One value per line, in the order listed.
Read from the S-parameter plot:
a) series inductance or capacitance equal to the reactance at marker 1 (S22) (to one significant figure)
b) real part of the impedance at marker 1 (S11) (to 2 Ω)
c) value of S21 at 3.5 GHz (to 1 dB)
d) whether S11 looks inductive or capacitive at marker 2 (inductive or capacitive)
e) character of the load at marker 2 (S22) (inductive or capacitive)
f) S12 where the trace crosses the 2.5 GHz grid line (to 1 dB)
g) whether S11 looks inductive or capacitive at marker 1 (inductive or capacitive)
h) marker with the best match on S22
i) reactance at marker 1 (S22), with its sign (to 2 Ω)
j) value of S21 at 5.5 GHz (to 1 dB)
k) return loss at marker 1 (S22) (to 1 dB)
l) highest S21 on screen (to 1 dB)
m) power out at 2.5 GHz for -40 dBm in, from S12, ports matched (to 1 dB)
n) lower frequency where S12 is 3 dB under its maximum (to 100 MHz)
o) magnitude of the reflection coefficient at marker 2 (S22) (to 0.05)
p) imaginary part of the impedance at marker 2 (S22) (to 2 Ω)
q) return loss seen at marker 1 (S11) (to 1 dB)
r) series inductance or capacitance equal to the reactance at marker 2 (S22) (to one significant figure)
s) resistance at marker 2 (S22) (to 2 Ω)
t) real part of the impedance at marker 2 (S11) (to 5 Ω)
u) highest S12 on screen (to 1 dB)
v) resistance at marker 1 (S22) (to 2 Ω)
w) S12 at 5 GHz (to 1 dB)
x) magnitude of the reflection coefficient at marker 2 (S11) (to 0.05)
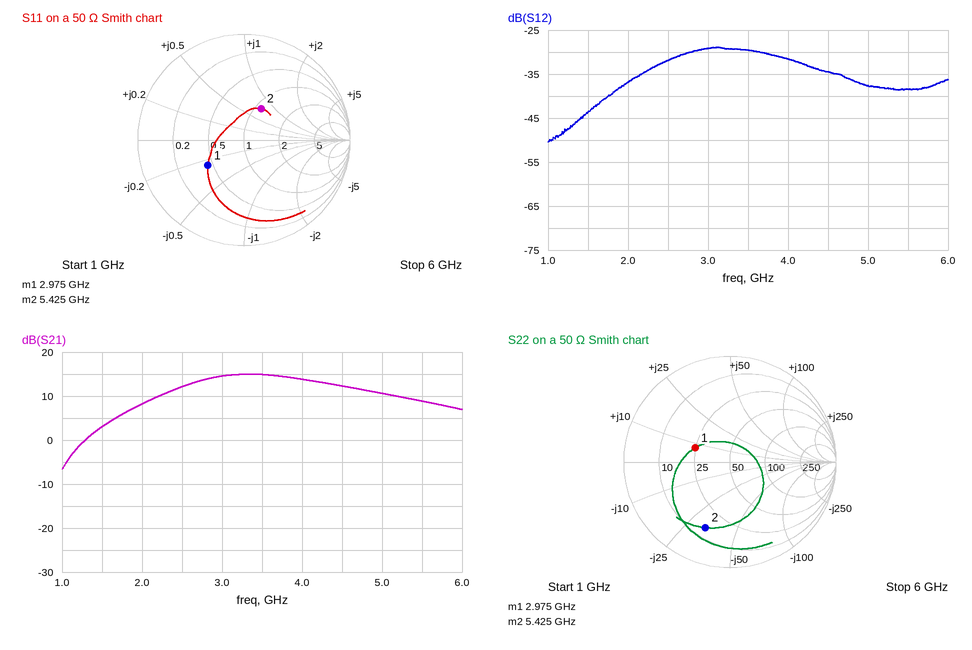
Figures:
400 pH
22 Ω
15 dB
inductive
capacitive
-32 dB
capacitive
marker 1
+8 Ω
9 dB
9 dB
15 dB
-72 dBm
2.5 GHz
0.65
-32 Ω
8 dB
900 fF
14 Ω
55 Ω
-29 dB
24 Ω
-38 dB
0.35
